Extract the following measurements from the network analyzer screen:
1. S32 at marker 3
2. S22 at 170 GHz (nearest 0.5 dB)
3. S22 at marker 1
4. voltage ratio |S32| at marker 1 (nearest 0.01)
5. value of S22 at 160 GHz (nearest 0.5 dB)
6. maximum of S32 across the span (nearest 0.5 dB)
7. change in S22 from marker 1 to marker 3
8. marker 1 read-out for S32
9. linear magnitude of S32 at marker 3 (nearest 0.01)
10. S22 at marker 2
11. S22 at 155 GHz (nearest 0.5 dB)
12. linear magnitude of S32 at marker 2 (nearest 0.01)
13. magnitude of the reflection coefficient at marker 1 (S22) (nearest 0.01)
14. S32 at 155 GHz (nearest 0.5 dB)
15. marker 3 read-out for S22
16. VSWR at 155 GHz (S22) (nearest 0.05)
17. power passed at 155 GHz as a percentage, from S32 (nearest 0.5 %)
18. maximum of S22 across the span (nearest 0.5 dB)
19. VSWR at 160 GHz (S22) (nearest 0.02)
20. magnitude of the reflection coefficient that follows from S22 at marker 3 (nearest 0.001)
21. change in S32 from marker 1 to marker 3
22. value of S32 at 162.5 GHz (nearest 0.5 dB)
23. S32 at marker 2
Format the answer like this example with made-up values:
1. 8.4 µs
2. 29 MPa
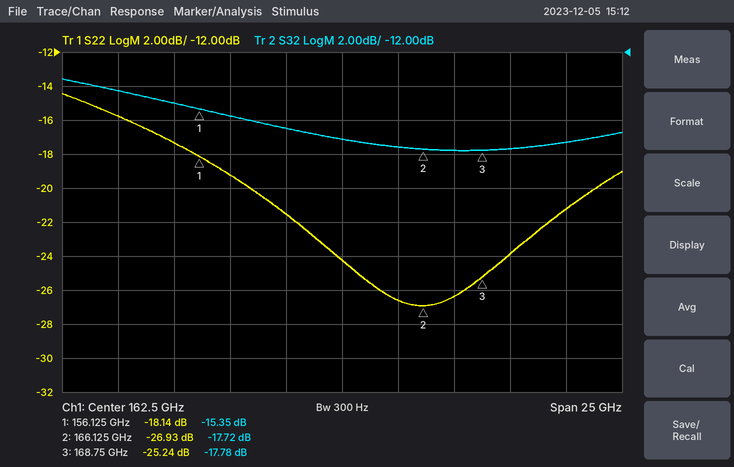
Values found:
1. -17.78 dB
2. -24.0 dB
3. -18.14 dB
4. 0.17
5. -21.5 dB
6. -13.5 dB
7. -7.10 dB
8. -15.35 dB
9. 0.13
10. -26.93 dB
11. -17.5 dB
12. 0.13
13. 0.12
14. -15.0 dB
15. -25.24 dB
16. 1.30
17. 3.0 %
18. -14.5 dB
19. 1.18
20. 0.055
21. -2.43 dB
22. -17.0 dB
23. -17.72 dB
